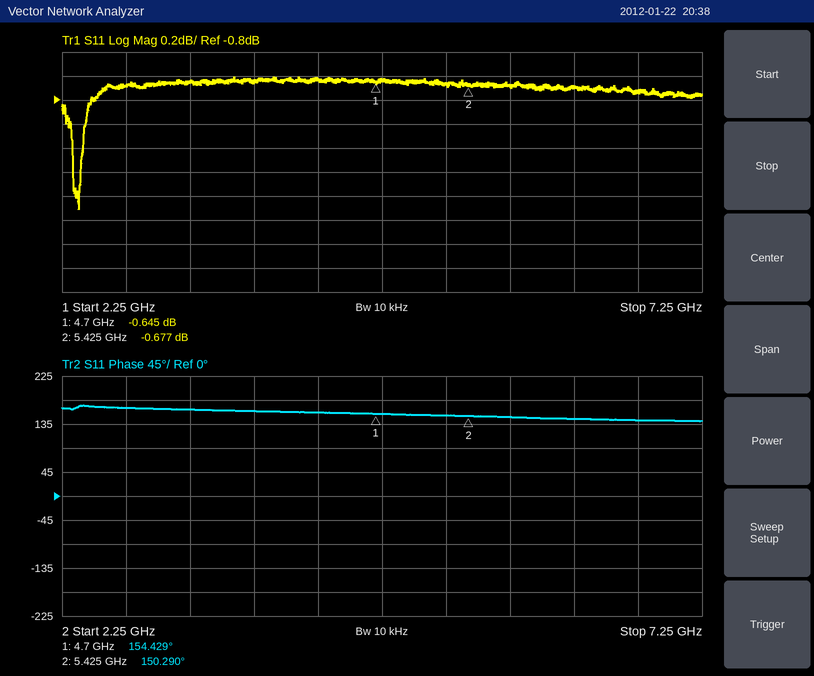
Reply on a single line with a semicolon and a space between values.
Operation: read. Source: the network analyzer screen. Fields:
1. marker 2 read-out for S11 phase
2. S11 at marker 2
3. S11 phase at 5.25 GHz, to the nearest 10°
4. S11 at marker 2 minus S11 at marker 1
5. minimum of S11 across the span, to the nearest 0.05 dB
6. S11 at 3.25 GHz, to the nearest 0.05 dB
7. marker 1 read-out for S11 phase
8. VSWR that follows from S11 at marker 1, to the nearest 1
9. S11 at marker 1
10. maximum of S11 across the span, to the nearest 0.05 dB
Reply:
150.290°; -0.677 dB; 150°; -0.032 dB; -1.70 dB; -0.65 dB; 154.429°; 27; -0.645 dB; -0.60 dB
